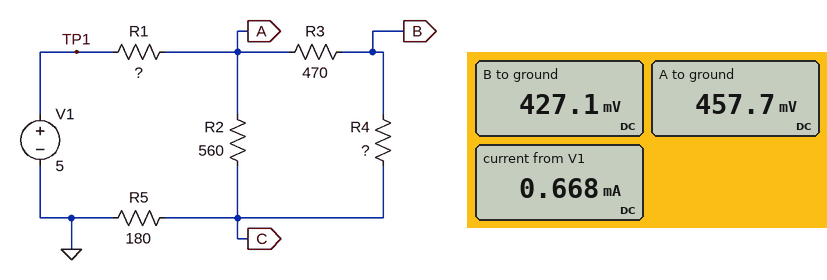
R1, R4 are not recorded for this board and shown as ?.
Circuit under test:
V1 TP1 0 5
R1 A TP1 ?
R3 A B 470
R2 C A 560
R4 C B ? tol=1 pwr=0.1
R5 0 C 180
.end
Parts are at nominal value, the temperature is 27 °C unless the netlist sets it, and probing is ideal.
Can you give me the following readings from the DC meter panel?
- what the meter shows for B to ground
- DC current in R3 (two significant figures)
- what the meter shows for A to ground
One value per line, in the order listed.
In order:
427.1 mV
65 µA
457.7 mV
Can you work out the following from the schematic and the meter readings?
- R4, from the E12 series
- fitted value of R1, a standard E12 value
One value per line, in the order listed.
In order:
4.7 kΩ
6.8 kΩ
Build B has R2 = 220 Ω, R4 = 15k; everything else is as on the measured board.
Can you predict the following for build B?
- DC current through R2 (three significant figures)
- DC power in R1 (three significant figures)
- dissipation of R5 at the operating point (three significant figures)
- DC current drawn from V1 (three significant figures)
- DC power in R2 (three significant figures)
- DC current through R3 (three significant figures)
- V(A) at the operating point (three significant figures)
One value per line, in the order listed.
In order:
685 µA
3.28 mW
86.9 µW
695 µA
103 µW
9.74 µA
276 mV
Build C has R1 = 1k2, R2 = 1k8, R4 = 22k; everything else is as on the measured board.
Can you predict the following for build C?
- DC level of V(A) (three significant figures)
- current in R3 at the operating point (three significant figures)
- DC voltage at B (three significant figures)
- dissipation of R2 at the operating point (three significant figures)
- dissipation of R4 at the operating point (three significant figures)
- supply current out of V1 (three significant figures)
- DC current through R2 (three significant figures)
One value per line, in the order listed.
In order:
3.03 V
122 µA
2.97 V
4.16 mW
326 µW
1.64 mA
1.52 mA
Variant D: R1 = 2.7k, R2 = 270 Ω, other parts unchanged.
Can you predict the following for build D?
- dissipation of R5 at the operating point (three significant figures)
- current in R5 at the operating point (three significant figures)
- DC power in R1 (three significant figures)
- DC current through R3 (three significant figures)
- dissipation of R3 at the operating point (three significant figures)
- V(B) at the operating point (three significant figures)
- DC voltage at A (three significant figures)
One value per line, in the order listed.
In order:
457 µW
1.59 mA
6.86 mW
79.1 µA
2.94 µW
659 mV
696 mV
